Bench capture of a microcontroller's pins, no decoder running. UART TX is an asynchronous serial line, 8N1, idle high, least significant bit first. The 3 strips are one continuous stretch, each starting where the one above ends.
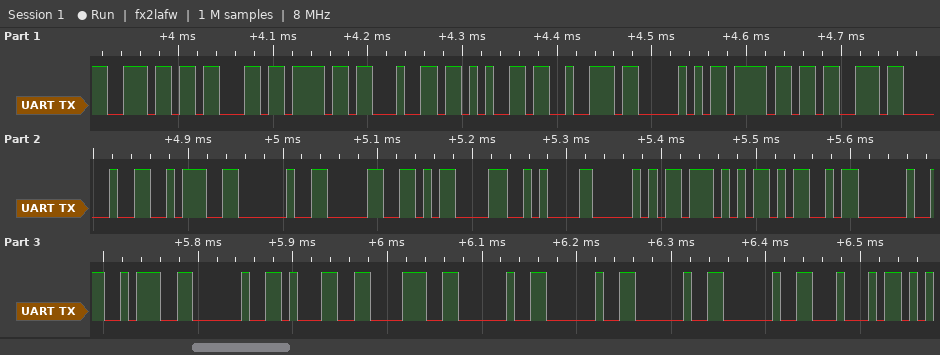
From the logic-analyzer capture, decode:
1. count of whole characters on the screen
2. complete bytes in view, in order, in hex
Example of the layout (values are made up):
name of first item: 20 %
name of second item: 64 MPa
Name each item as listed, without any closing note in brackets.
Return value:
count of whole characters on the screen: 28
complete bytes in view, in order, in hex: 6E 63 6F 64 65 72 50 6F 73 20 3A 20 30 0D 0A 50 57 4D 20 3A 20 31 38 20 20 20 20 44
